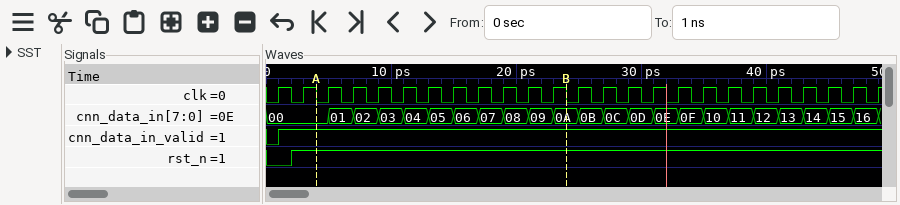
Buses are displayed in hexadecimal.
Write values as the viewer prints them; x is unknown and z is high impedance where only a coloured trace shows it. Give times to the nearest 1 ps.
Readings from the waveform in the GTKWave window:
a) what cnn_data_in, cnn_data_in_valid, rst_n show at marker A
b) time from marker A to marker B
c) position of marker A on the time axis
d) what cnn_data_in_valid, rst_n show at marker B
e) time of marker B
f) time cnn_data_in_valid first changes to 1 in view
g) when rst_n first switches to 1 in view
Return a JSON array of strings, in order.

["cnn_data_in=00, cnn_data_in_valid=1, rst_n=1", "20 ps", "4 ps", "cnn_data_in_valid=1, rst_n=1", "24 ps", "1 ps", "2 ps"]
